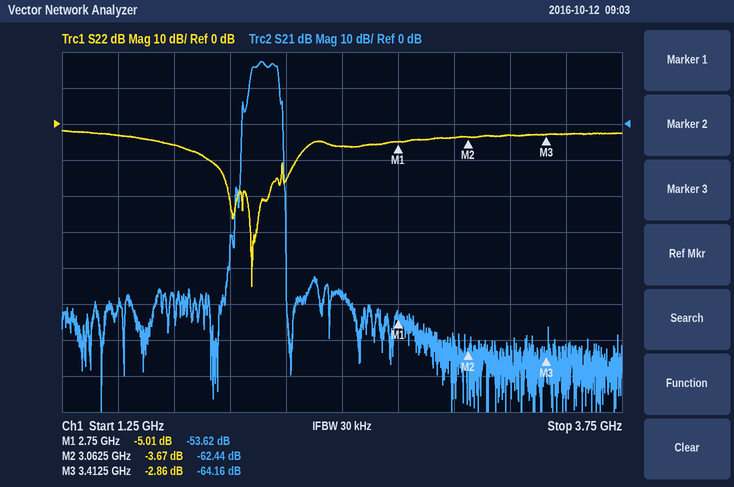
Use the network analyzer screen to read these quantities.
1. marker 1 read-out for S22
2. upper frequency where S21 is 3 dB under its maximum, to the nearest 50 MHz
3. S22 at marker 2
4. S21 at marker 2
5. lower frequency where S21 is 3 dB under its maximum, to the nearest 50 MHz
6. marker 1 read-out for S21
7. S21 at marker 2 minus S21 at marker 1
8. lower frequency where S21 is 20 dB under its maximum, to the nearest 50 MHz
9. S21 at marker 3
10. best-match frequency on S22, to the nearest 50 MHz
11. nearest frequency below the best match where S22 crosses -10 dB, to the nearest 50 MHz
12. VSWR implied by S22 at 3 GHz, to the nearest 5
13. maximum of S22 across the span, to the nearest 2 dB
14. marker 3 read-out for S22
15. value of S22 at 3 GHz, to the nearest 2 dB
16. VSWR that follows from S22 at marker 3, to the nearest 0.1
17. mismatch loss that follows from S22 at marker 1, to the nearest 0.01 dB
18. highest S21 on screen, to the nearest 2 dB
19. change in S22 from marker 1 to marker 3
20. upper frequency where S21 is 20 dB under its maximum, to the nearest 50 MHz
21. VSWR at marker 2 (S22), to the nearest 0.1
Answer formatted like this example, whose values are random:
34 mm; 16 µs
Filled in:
-5.01 dB; 2.20 GHz; -3.67 dB; -62.44 dB; 2.10 GHz; -53.62 dB; -8.82 dB; 2.05 GHz; -64.16 dB; 2.10 GHz; 1.90 GHz; 5; -2 dB; -2.86 dB; -4 dB; 6.1; 1.65 dB; 18 dB; 2.15 dB; 2.25 GHz; 4.8
